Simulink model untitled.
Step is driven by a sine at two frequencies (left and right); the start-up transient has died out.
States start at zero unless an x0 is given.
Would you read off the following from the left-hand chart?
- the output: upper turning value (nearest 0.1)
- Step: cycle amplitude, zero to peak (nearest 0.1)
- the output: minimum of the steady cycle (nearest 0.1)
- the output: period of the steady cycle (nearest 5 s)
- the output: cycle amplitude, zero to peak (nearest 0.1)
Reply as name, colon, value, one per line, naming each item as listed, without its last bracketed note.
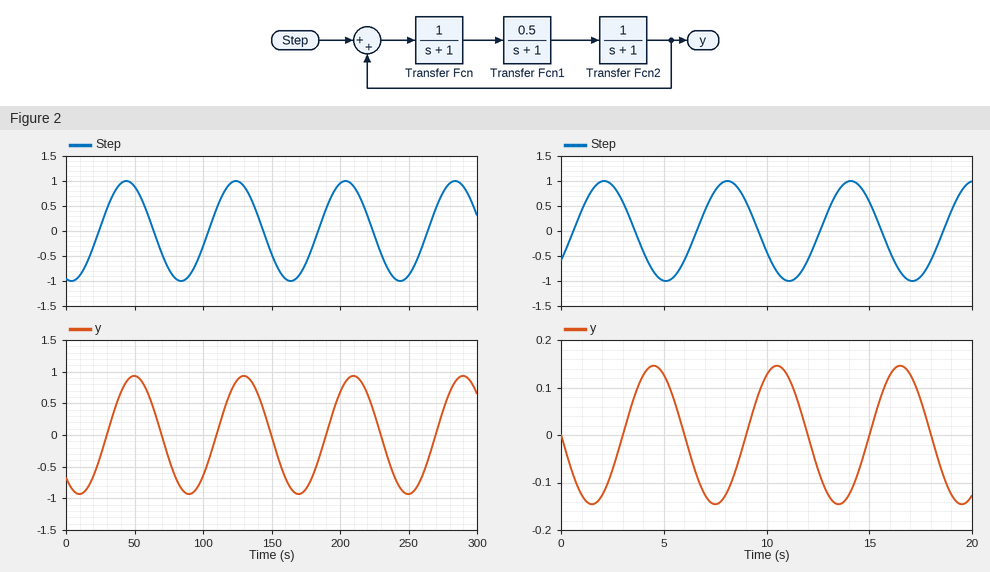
the output: upper turning value: 0.9
Step: cycle amplitude, zero to peak: 1.0
the output: minimum of the steady cycle: -0.9
the output: period of the steady cycle: 80 s
the output: cycle amplitude, zero to peak: 0.9
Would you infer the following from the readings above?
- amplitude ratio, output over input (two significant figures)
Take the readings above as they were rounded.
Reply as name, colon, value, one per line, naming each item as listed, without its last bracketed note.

amplitude ratio, output over input: 0.90
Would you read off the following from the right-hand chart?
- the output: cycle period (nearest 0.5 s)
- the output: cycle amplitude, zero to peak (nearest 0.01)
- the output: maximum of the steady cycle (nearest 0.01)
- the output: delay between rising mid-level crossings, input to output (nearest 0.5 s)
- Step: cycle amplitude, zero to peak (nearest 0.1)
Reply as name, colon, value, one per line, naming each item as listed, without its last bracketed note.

the output: cycle period: 6.0 s
the output: cycle amplitude, zero to peak: 0.15
the output: maximum of the steady cycle: 0.15
the output: delay between rising mid-level crossings, input to output: 2.5 s
Step: cycle amplitude, zero to peak: 1.0
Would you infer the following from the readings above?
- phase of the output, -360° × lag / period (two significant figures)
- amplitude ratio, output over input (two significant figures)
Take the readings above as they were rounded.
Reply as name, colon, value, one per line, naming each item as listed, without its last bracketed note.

phase of the output, -360° × lag / period: -150°
amplitude ratio, output over input: 0.15
